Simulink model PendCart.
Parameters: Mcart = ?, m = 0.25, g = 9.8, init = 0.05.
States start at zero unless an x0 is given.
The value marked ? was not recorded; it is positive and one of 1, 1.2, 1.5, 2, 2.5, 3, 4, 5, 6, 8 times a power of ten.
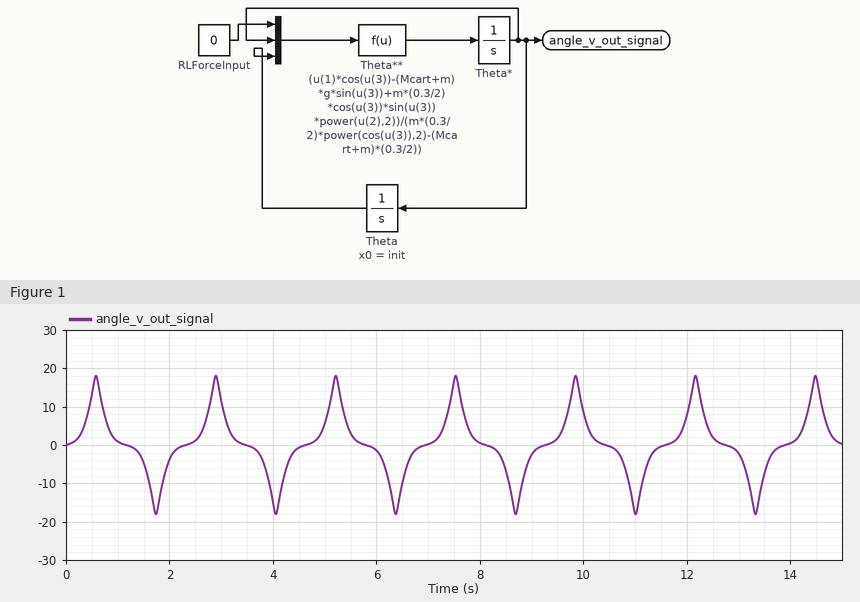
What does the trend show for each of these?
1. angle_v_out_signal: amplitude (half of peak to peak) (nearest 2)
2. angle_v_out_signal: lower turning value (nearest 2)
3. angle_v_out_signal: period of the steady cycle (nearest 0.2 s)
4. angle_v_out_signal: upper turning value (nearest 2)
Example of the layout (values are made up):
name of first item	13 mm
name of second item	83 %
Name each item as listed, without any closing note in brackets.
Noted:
angle_v_out_signal: amplitude (half of peak to peak)	18
angle_v_out_signal: lower turning value	-18
angle_v_out_signal: period of the steady cycle	2.4 s
angle_v_out_signal: upper turning value	18
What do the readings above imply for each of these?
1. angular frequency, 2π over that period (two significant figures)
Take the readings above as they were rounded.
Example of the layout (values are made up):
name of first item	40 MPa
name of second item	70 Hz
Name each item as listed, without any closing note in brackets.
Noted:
angular frequency, 2π over that period	2.6 rad/s
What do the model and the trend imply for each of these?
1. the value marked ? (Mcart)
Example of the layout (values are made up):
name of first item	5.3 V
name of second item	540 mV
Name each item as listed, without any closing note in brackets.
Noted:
the value marked ?	1
